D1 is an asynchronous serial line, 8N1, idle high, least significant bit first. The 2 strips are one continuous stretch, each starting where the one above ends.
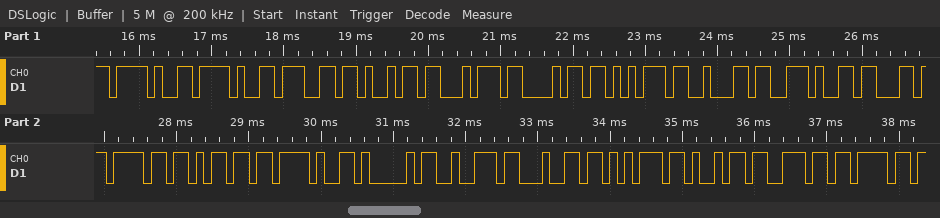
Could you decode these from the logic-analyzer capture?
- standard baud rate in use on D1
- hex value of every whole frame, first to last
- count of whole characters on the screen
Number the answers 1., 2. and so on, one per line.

1. 9600 baud
2. 0x2F 0x2F 0x67 0x69 0x74 0x68 0x75 0x62 0x2E 0x63 0x6F 0x6D 0x2F 0x41 0x72 0x64 0x75 0x69 0x6E 0x6F
3. 20
